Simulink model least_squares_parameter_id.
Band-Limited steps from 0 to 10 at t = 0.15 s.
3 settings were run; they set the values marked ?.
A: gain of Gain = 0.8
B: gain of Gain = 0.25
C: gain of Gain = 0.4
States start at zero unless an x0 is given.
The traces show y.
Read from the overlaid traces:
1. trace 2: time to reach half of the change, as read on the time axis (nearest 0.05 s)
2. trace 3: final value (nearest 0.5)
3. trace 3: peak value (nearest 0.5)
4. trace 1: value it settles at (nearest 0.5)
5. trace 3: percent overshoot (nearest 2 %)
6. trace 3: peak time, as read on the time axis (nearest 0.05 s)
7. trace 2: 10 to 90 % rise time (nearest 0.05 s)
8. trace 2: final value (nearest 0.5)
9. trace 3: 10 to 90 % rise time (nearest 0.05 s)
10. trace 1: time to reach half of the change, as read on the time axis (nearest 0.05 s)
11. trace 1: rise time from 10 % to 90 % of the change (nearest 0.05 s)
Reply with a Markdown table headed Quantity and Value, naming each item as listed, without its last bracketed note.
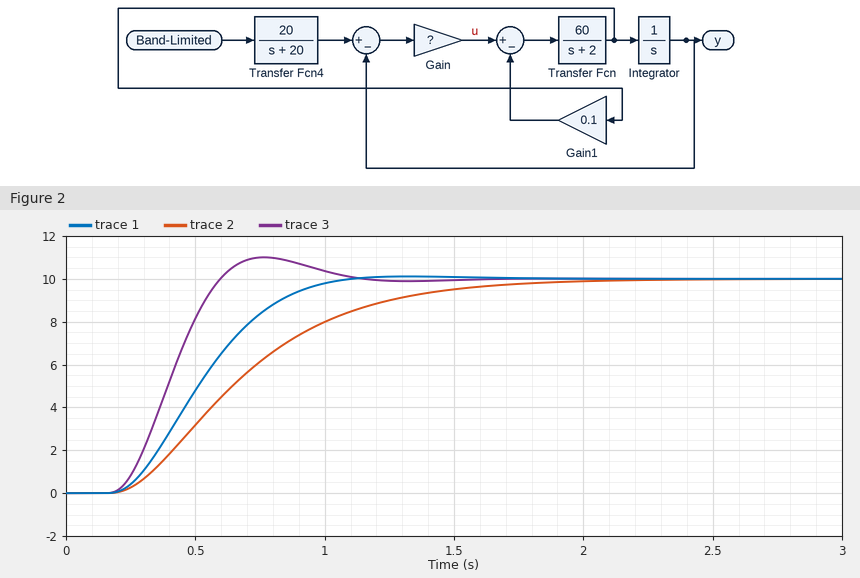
| Quantity | Value |
|---|---|
| trace 2: time to reach half of the change, as read on the time axis | 0.65 s |
| trace 3: final value | 10.0 |
| trace 3: peak value | 11.0 |
| trace 1: value it settles at | 10.0 |
| trace 3: percent overshoot | 10 % |
| trace 3: peak time, as read on the time axis | 0.75 s |
| trace 2: 10 to 90 % rise time | 0.90 s |
| trace 2: final value | 10.0 |
| trace 3: 10 to 90 % rise time | 0.30 s |
| trace 1: time to reach half of the change, as read on the time axis | 0.50 s |
| trace 1: rise time from 10 % to 90 % of the change | 0.55 s |
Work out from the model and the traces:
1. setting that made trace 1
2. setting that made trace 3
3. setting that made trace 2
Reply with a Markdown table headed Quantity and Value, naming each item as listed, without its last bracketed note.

| Quantity | Value |
|---|---|
| setting that made trace 1 | C |
| setting that made trace 3 | A |
| setting that made trace 2 | B |
